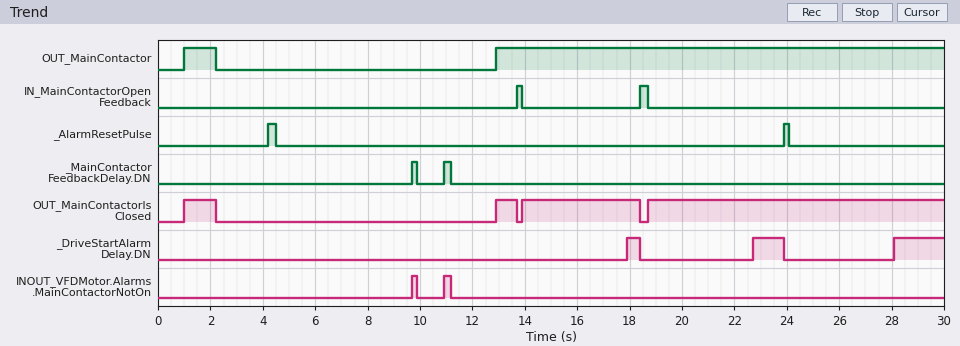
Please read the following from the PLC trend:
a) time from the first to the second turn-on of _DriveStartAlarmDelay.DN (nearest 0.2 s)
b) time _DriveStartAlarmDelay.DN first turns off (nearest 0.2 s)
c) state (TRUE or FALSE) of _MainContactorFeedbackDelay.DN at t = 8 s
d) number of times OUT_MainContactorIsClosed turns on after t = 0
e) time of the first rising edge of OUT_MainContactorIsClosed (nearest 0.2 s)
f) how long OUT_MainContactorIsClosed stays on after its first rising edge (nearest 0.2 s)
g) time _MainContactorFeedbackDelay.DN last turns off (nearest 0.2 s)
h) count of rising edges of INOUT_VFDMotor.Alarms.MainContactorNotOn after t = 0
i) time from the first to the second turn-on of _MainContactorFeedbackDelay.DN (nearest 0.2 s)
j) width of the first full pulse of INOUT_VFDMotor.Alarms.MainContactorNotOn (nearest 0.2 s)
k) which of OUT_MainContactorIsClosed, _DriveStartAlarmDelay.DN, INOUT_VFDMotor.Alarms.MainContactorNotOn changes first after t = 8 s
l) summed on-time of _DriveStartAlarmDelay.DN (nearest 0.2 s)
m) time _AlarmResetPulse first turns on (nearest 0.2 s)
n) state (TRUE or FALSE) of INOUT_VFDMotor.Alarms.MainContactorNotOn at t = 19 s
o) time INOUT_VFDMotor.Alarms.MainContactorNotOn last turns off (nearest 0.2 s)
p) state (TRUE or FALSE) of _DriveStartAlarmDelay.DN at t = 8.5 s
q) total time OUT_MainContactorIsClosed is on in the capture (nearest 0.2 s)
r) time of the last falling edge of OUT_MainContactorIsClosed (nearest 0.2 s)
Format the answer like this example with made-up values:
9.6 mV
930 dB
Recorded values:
4.8 s
18.4 s
FALSE
4
1.0 s
1.2 s
11.2 s
2
1.2 s
0.2 s
INOUT_VFDMotor.Alarms.MainContactorNotOn
3.6 s
4.2 s
FALSE
11.2 s
FALSE
17.8 s
18.4 s
